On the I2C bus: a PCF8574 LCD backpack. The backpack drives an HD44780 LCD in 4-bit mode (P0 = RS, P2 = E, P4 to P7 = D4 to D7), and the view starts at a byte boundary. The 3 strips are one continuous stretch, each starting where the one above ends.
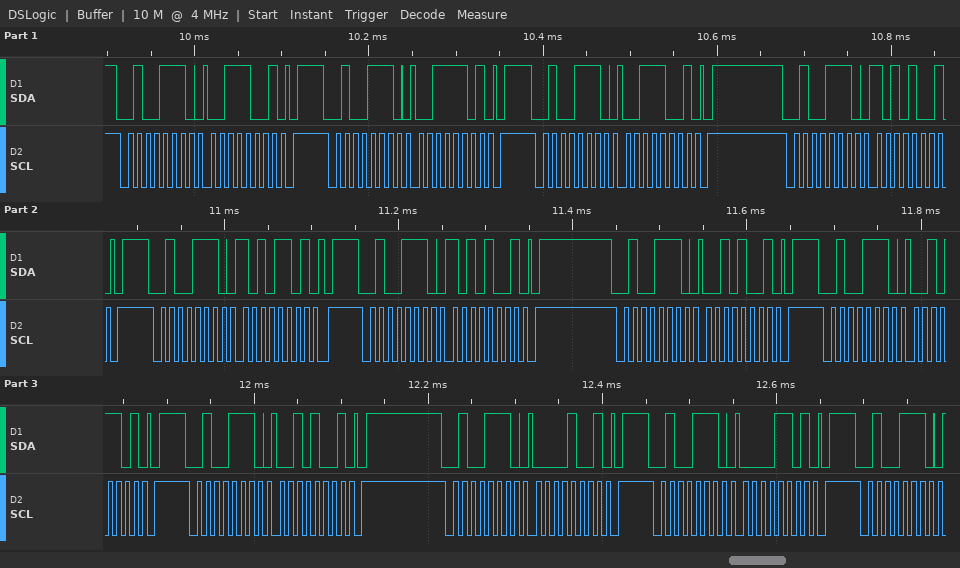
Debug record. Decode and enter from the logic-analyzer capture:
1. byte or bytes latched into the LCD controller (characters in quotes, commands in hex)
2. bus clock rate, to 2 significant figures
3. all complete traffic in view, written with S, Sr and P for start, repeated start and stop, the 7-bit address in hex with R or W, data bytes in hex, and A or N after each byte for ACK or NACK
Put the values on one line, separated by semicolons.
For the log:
':'; 100 kHz; S 27W A 39 A P S 27W A 3D A P S 27W A 39 A P S 27W A A9 A P S 27W A AD A P S 27W A A9 A P S 27W A 29 A P S 27W A 2D A P S 27W A 29 A P S 27W A 09 A P S 27W A 0D A P S 27W A
